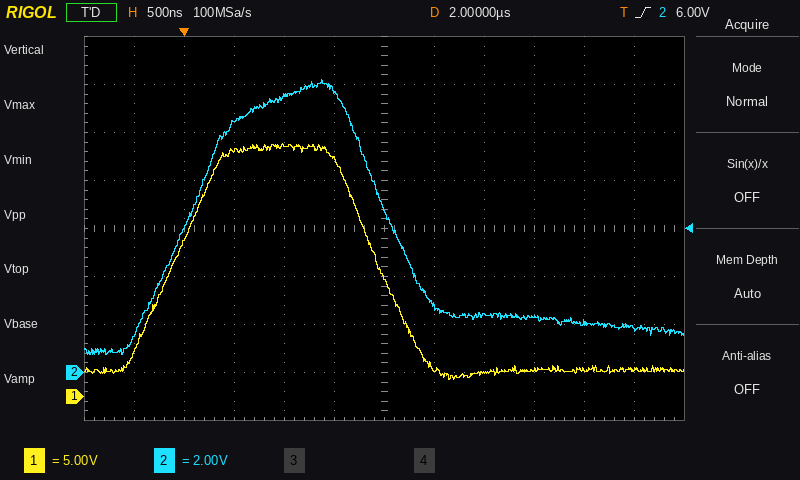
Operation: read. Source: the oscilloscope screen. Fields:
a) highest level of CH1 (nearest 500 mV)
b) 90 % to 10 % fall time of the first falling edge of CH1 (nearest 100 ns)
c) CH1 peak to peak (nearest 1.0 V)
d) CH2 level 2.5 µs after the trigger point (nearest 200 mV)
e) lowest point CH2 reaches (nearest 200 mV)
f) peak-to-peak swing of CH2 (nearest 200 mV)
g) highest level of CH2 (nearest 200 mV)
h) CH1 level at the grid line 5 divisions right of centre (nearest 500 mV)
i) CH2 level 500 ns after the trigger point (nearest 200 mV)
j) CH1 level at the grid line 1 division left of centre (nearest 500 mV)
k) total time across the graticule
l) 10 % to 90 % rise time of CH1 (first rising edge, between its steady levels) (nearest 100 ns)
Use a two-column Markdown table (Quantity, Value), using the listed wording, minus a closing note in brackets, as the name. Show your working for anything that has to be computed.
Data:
| Quantity | Value |
|---|---|
| highest level of CH1 | 26.5 V |
| 90 % to 10 % fall time of the first falling edge of CH1 | 800 ns |
| CH1 peak to peak | 25.0 V |
| CH2 level 2.5 µs after the trigger point | 2.8 V |
| lowest point CH2 reaches | 800 mV |
| peak-to-peak swing of CH2 | 12.2 V − (800 mV) = 11.4 V |
| highest level of CH2 | 12.2 V |
| CH1 level at the grid line 5 divisions right of centre | 3.0 V |
| CH2 level 500 ns after the trigger point | 10.4 V |
| CH1 level at the grid line 1 division left of centre | 24.5 V |
| total time across the graticule | 6 µs |
| 10 % to 90 % rise time of CH1 (first rising edge, between its steady levels) | 800 ns |
